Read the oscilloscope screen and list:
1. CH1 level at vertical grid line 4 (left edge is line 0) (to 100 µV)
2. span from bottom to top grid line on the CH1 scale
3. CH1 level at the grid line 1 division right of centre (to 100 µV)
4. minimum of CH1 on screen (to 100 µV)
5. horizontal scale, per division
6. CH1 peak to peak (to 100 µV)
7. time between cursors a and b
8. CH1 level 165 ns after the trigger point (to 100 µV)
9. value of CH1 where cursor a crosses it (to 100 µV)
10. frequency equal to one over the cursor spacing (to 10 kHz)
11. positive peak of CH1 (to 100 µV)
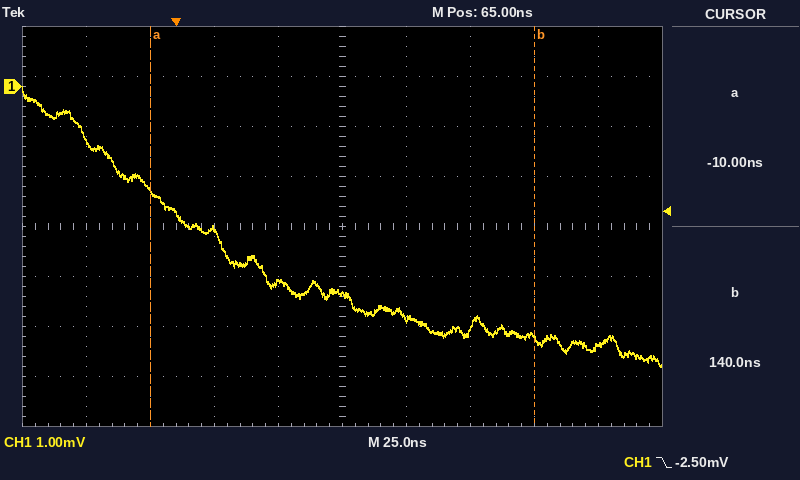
-3.9 mV
8 mV
-4.6 mV
-5.6 mV
25 ns
5.6 mV
150.0 ns
-5.2 mV
-2.1 mV
6.67 MHz
0.0 mV
